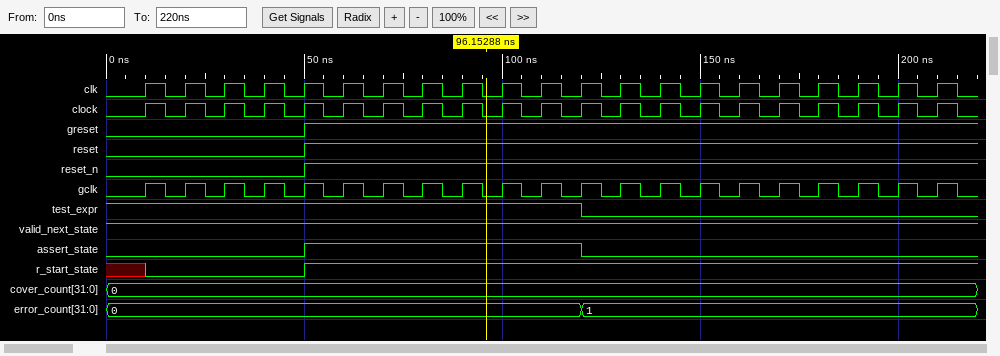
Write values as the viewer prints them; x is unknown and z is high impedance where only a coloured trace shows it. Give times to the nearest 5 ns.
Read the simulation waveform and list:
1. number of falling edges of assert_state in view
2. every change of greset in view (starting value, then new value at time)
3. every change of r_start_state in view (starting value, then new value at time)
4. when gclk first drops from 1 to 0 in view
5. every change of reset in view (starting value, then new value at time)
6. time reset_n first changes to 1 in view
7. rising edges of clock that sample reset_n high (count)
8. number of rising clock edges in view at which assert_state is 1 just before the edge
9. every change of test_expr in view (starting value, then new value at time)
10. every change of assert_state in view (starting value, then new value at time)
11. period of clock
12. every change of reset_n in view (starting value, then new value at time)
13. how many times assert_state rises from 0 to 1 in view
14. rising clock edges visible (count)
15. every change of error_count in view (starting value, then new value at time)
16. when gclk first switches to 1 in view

1
0, 1 at 50 ns
x, 0 at 10 ns, 1 at 50 ns
15 ns
0, 1 at 50 ns
50 ns
16
7
1, 0 at 120 ns
0, 1 at 50 ns, 0 at 120 ns
10 ns
0, 1 at 50 ns
1
21
0, 1 at 120 ns
10 ns
